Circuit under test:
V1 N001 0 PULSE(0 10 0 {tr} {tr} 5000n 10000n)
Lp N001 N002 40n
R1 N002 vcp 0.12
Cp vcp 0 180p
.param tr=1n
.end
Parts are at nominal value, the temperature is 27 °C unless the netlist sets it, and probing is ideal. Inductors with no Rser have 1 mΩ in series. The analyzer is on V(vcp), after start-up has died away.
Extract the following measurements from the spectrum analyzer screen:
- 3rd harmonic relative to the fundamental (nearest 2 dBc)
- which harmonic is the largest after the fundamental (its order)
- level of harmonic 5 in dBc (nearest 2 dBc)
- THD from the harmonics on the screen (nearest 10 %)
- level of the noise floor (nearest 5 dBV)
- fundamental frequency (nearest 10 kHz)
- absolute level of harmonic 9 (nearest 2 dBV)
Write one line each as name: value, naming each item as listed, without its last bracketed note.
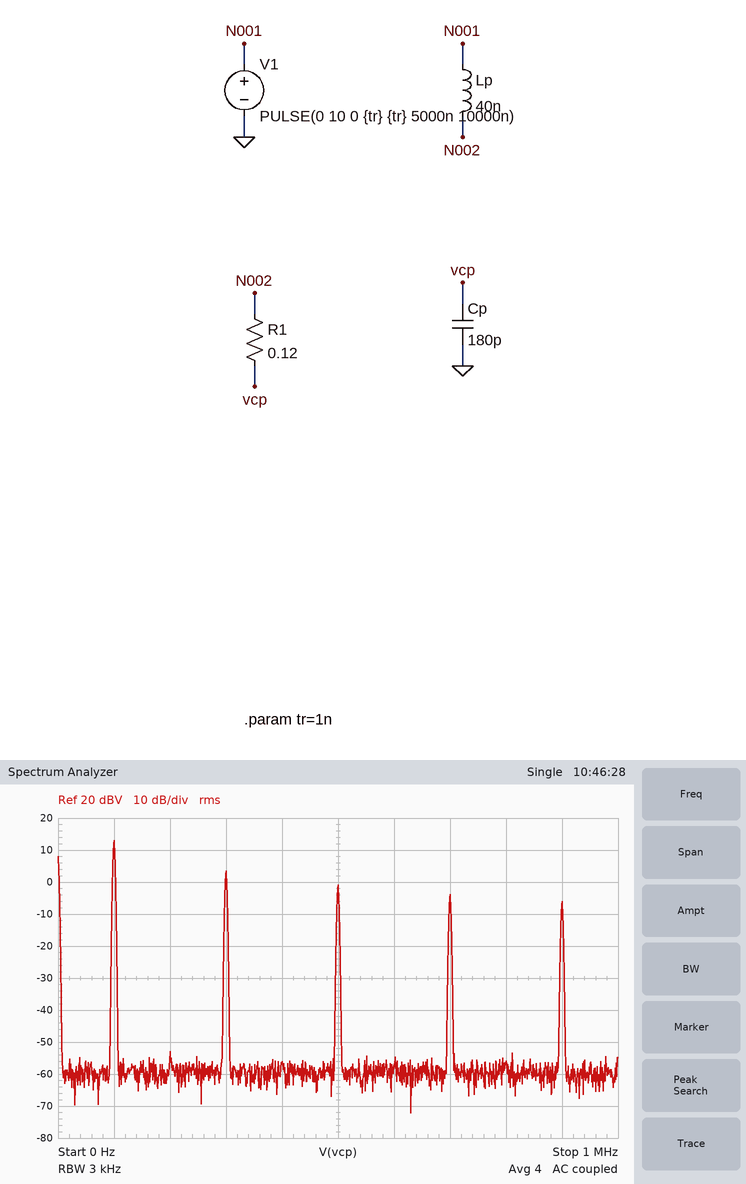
3rd harmonic relative to the fundamental: -10 dBc
which harmonic is the largest after the fundamental: 3
level of harmonic 5 in dBc: -14 dBc
THD from the harmonics on the screen: 40 %
level of the noise floor: -60 dBV
fundamental frequency: 100 kHz
absolute level of harmonic 9: -6 dBV
